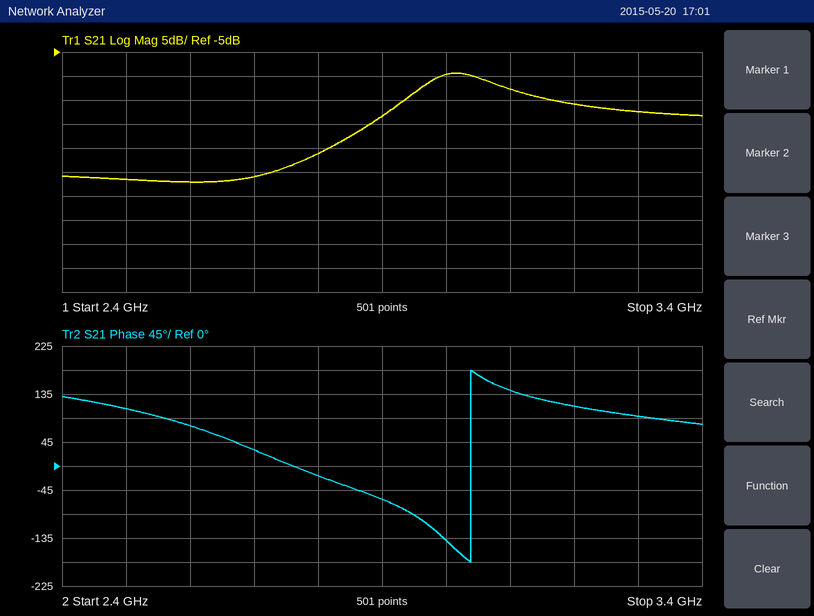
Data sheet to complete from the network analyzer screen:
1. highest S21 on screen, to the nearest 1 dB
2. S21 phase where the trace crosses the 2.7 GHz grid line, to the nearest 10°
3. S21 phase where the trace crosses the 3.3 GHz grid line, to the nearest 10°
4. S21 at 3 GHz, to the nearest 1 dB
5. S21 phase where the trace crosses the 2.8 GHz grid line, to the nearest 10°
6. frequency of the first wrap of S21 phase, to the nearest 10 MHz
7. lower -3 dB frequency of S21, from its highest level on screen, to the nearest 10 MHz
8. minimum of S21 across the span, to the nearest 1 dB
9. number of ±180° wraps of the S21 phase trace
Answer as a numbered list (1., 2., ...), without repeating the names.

1. -9 dB
2. 30°
3. 90°
4. -10 dB
5. -20°
6. 3.04 GHz
7. 2.96 GHz
8. -32 dB
9. 1
